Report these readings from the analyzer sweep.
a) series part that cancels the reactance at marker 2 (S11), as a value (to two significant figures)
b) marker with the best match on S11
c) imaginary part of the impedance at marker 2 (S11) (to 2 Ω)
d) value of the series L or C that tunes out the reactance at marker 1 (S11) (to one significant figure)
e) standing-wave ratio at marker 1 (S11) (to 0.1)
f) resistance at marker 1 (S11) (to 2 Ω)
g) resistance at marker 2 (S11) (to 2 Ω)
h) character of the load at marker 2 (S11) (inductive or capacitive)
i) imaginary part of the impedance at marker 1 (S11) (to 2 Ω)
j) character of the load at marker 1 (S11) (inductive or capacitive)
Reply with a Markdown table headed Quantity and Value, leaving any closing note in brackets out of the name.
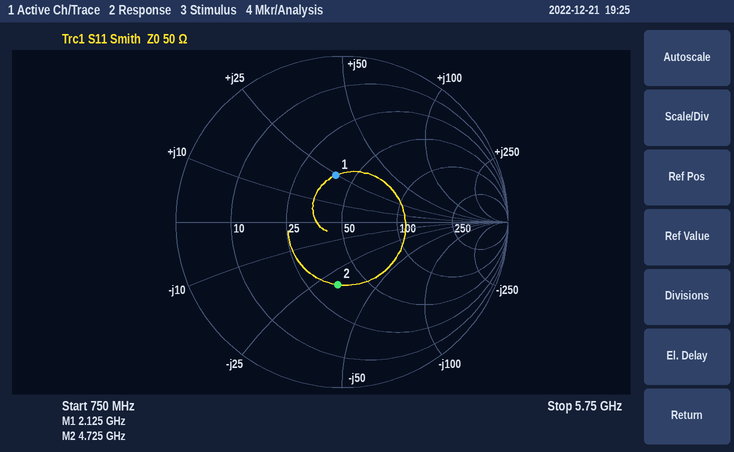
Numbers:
| Quantity | Value |
|---|---|
| series part that cancels the reactance at marker 2 (S11), as a value | 1.1 nH |
| marker with the best match on S11 | marker 1 |
| imaginary part of the impedance at marker 2 (S11) | -32 Ω |
| value of the series L or C that tunes out the reactance at marker 1 (S11) | 3 pF |
| standing-wave ratio at marker 1 (S11) | 1.8 |
| resistance at marker 1 (S11) | 40 Ω |
| resistance at marker 2 (S11) | 36 Ω |
| character of the load at marker 2 (S11) | capacitive |
| imaginary part of the impedance at marker 1 (S11) | +24 Ω |
| character of the load at marker 1 (S11) | inductive |
